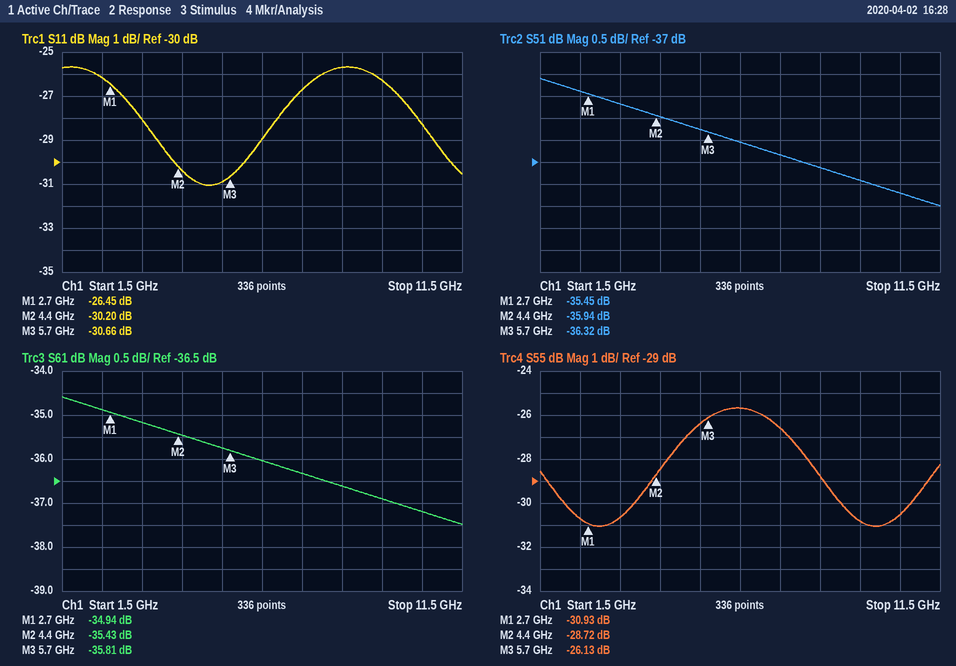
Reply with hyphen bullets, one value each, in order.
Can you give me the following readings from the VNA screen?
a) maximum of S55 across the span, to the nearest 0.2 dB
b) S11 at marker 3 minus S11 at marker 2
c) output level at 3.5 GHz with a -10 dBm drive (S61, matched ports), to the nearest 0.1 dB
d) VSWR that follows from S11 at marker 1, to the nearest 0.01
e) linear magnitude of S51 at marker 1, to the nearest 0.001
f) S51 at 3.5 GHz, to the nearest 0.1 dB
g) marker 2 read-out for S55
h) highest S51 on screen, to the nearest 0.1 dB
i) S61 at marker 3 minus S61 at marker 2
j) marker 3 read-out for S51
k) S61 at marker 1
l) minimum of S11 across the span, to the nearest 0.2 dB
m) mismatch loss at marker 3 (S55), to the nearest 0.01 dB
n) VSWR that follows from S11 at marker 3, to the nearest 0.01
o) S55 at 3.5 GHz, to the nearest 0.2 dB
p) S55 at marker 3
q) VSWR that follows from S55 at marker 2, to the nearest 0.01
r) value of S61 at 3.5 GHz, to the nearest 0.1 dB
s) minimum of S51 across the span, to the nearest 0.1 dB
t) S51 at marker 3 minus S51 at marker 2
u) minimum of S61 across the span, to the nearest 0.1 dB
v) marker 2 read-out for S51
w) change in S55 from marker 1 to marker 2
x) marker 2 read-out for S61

- -25.6 dB
- -0.46 dB
- -45.2 dBm
- 1.10
- 0.017
- -35.7 dB
- -28.72 dB
- -35.1 dB
- -0.38 dB
- -36.32 dB
- -34.94 dB
- -31.0 dB
- 0.01 dB
- 1.06
- -30.6 dB
- -26.13 dB
- 1.08
- -35.2 dB
- -38.0 dB
- -0.38 dB
- -37.5 dB
- -35.94 dB
- 2.21 dB
- -35.43 dB
